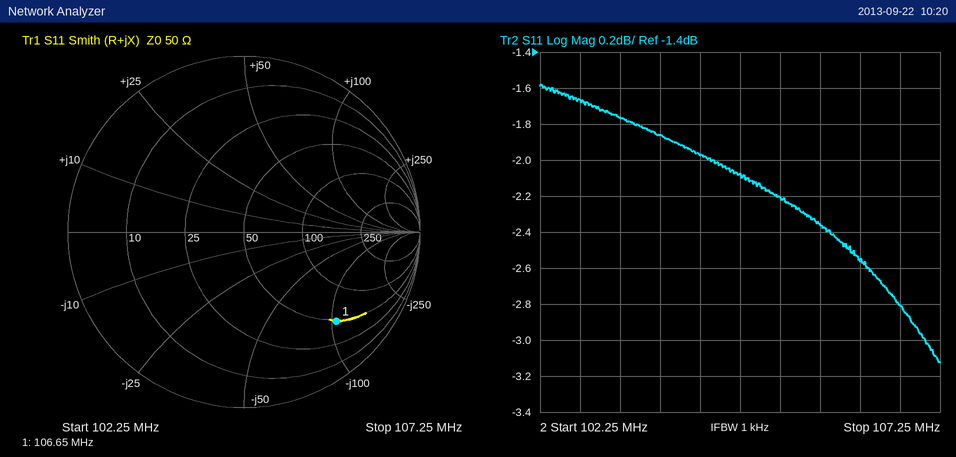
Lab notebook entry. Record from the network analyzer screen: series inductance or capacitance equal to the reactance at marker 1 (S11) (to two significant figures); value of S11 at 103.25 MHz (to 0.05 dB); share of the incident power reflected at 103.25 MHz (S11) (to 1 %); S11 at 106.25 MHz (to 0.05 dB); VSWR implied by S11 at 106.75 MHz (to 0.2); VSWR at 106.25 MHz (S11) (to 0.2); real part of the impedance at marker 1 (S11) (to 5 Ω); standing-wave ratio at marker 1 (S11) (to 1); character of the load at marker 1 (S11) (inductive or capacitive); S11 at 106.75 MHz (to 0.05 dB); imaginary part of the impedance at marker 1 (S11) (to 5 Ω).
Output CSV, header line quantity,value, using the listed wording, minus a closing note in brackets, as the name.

quantity,value
series inductance or capacitance equal to the reactance at marker 1 (S11),14 pF
value of S11 at 103.25 MHz,-1.75 dB
share of the incident power reflected at 103.25 MHz (S11),67 %
S11 at 106.25 MHz,-2.55 dB
VSWR implied by S11 at 106.75 MHz,6.2
VSWR at 106.25 MHz (S11),6.8
real part of the impedance at marker 1 (S11),50 Ω
standing-wave ratio at marker 1 (S11),6
character of the load at marker 1 (S11),capacitive
S11 at 106.75 MHz,-2.80 dB
imaginary part of the impedance at marker 1 (S11),-105 Ω
